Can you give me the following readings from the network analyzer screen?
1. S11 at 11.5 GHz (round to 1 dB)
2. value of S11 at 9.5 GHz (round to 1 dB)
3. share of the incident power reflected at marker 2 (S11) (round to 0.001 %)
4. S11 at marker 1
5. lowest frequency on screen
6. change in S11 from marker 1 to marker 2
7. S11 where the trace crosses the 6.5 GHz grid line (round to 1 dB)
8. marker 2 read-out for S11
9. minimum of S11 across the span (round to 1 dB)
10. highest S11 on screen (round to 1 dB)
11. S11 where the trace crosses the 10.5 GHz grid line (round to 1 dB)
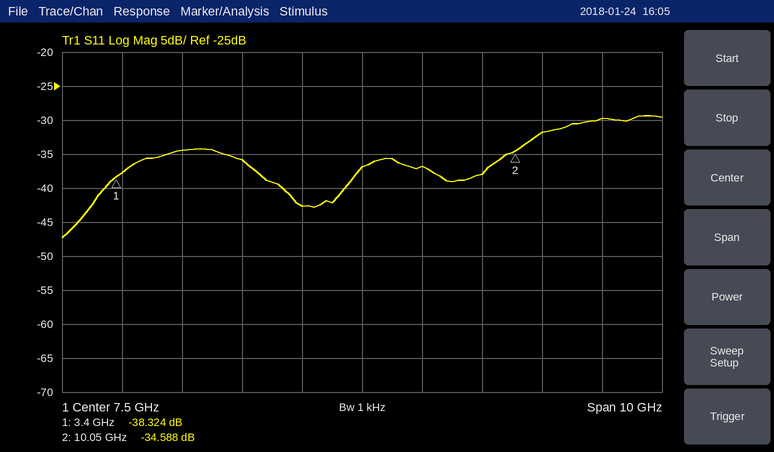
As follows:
-30 dB
-38 dB
0.035 %
-38.324 dB
2.5 GHz
3.736 dB
-43 dB
-34.588 dB
-47 dB
-29 dB
-32 dB
